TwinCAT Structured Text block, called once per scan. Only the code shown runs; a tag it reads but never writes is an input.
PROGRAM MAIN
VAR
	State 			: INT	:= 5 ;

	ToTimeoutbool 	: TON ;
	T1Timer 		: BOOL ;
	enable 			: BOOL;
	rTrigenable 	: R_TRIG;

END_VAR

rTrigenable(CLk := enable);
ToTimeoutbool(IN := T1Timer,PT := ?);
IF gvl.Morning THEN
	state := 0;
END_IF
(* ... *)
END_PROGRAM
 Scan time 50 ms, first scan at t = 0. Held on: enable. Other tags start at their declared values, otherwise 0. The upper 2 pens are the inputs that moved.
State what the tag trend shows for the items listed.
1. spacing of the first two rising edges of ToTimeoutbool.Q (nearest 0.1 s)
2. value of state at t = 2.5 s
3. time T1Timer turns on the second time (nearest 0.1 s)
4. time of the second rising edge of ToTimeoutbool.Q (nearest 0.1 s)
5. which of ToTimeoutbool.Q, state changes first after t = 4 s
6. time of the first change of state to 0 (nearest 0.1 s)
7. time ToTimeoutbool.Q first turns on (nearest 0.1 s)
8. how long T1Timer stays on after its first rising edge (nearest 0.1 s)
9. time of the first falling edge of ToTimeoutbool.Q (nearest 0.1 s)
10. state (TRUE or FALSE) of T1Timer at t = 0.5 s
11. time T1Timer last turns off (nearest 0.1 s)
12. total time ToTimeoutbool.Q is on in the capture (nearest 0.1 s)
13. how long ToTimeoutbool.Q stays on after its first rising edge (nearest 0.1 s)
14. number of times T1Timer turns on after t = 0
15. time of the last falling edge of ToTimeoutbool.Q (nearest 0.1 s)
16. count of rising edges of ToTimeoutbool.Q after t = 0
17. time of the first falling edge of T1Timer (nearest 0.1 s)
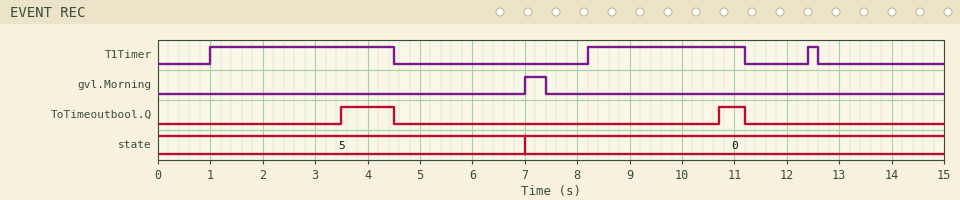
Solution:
7.2 s
5
8.2 s
10.7 s
ToTimeoutbool.Q
7.0 s
3.5 s
3.5 s
4.5 s
FALSE
12.6 s
1.5 s
1.0 s
3
11.2 s
2
4.5 s
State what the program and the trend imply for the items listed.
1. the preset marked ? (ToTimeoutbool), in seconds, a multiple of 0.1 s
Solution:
2.5 s
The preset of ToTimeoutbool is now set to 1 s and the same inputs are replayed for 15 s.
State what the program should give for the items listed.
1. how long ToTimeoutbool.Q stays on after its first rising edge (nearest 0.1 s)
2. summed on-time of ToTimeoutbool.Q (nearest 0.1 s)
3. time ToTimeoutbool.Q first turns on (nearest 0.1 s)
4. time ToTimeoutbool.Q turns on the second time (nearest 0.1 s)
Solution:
2.5 s
4.5 s
2.0 s
9.2 s
